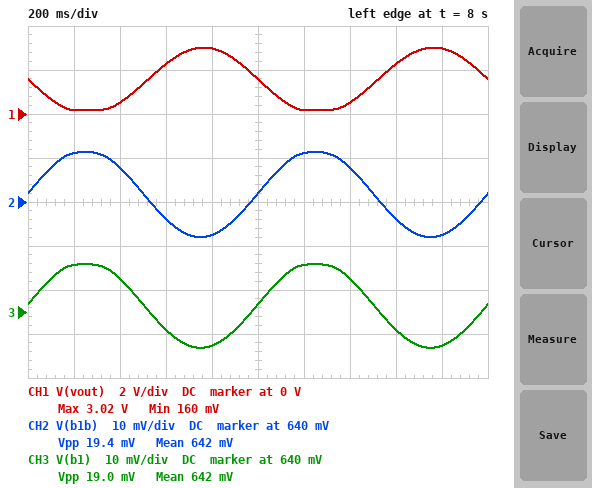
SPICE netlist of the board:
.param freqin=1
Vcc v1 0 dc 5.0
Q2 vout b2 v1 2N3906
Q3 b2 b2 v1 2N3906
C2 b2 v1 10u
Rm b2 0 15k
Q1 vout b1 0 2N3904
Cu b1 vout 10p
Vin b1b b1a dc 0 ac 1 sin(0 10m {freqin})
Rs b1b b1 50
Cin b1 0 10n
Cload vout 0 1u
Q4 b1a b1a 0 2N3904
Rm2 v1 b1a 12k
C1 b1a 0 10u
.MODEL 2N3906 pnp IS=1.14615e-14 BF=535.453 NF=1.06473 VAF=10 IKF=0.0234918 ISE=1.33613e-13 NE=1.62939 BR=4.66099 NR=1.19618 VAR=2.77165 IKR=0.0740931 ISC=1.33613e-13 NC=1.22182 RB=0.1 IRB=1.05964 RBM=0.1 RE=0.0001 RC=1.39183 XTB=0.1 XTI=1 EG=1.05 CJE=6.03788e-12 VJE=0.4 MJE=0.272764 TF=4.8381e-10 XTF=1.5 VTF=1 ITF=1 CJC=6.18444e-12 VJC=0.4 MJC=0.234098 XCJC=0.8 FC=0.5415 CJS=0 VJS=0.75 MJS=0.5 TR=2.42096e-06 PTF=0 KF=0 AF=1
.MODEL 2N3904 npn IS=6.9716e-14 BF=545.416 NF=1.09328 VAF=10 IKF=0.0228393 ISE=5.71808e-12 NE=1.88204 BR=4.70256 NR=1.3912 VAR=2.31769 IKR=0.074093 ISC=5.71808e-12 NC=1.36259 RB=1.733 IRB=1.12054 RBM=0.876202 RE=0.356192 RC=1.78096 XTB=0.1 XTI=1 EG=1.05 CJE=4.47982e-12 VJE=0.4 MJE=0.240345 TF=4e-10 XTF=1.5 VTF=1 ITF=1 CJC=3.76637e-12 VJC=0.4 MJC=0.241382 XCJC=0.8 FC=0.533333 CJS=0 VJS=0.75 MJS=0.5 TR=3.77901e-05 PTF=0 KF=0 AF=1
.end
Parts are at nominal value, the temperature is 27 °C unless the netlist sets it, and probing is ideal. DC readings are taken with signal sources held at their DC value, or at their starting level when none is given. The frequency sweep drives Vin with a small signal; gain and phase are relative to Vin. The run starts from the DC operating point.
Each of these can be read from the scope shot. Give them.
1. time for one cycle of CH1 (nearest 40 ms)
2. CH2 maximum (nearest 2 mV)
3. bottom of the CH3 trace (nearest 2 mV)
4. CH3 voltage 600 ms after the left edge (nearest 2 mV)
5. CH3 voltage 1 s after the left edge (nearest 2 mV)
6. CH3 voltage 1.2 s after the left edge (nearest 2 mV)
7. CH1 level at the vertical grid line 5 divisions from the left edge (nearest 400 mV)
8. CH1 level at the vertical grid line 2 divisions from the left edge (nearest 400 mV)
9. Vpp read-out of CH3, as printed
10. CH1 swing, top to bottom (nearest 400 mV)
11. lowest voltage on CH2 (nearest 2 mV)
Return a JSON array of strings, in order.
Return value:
["1.00 s", "652 mV", "632 mV", "636 mV", "642 mV", "650 mV", "1.6 V", "400 mV", "19.0 mV", "2.8 V", "632 mV"]
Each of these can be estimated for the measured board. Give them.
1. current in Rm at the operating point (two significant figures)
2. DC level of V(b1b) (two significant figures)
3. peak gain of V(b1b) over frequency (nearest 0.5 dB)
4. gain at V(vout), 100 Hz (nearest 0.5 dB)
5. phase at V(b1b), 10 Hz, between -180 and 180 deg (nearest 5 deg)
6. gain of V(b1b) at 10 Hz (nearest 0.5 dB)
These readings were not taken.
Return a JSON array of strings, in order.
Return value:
["290 µA", "640 mV", "0 dB", "26.5 dB", "0 deg", "0 dB"]
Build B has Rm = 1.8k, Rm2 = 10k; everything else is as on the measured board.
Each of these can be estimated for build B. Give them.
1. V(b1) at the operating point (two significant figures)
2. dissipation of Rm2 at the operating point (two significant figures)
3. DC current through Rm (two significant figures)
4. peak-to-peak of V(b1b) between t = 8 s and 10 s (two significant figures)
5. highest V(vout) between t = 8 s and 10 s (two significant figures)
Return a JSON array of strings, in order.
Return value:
["650 mV", "1.9 mW", "2.4 mA", "20 mV", "5.0 V"]
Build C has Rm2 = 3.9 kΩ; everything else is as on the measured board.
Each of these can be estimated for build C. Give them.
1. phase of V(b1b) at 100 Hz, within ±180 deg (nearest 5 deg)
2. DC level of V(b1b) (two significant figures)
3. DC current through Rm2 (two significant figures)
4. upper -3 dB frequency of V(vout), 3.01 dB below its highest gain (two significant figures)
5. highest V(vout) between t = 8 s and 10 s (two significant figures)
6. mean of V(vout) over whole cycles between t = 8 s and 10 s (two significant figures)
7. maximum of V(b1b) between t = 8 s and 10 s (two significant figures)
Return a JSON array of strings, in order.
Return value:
["5 deg", "670 mV", "1.1 mA", "1.8 kHz", "70 mV", "56 mV", "680 mV"]
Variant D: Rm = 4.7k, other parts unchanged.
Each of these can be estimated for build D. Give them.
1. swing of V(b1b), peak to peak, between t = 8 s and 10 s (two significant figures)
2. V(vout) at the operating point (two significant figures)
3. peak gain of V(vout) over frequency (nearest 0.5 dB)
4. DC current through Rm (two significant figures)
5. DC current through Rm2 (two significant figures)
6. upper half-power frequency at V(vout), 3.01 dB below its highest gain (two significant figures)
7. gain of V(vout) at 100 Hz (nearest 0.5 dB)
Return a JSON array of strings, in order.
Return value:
["20 mV", "5.0 V", "9.5 dB", "920 µA", "360 µA", "1.3 kHz", "8.5 dB"]
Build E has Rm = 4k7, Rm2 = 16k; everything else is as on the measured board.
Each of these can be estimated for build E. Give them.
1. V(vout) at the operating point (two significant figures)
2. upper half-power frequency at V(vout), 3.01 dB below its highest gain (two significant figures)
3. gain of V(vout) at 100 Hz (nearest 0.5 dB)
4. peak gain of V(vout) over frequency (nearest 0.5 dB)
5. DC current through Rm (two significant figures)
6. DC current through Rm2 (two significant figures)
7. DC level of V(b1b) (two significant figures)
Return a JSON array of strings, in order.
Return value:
["5.0 V", "1.7 kHz", "3.0 dB", "4.5 dB", "920 µA", "270 µA", "630 mV"]
